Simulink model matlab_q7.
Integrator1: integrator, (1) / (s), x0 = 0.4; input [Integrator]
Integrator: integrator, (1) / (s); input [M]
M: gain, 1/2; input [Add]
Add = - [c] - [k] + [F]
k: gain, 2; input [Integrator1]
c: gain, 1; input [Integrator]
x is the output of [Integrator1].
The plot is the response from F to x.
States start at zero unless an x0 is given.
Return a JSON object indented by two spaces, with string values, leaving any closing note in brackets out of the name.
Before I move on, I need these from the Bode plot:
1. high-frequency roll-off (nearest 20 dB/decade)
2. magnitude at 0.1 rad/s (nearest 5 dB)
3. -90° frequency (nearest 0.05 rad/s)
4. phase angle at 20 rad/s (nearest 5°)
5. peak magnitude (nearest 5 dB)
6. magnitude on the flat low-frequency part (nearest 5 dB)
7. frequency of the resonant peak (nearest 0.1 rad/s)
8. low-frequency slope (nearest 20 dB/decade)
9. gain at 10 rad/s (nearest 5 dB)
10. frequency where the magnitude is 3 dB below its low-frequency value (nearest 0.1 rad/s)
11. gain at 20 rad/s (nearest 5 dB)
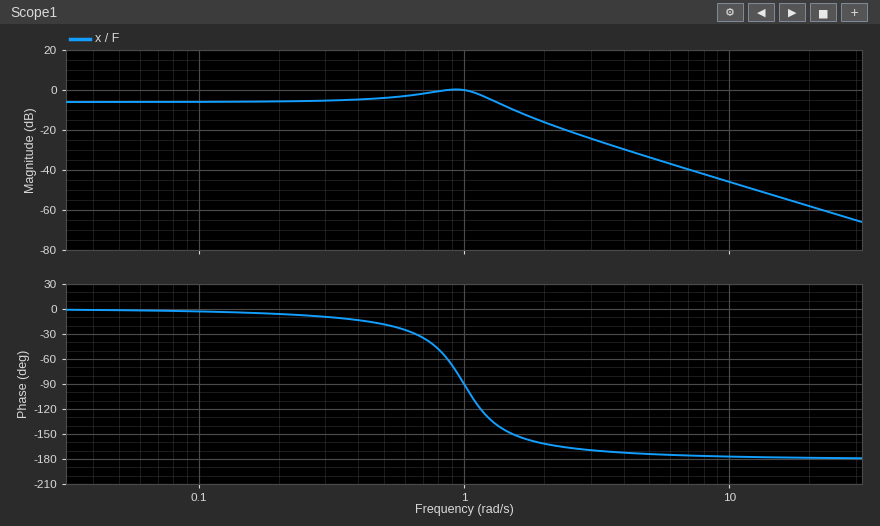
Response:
{
  "high-frequency roll-off": "-40 dB/decade",
  "magnitude at 0.1 rad/s": "-5 dB",
  "-90° frequency": "1.00 rad/s",
  "phase angle at 20 rad/s": "-180°",
  "peak magnitude": "0 dB",
  "magnitude on the flat low-frequency part": "-5 dB",
  "frequency of the resonant peak": "0.9 rad/s",
  "low-frequency slope": "0 dB/decade",
  "gain at 10 rad/s": "-45 dB",
  "frequency where the magnitude is 3 dB below its low-frequency value": "1.5 rad/s",
  "gain at 20 rad/s": "-60 dB"
}
